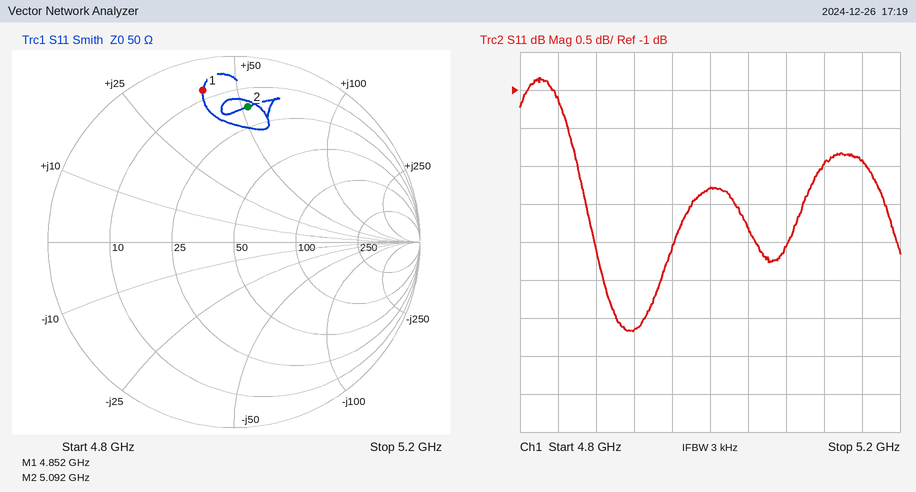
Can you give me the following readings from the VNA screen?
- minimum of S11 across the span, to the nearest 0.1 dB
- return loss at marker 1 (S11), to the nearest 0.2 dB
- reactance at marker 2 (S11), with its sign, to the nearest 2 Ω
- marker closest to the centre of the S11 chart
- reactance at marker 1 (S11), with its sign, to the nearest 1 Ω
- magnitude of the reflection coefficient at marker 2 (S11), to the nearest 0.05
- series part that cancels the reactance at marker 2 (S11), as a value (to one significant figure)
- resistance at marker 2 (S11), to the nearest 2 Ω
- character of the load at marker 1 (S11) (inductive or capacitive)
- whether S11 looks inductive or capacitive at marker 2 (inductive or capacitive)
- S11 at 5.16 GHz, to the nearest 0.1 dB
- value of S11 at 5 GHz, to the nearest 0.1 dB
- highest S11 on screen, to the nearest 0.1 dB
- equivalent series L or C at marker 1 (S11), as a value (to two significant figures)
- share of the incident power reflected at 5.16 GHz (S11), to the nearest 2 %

-4.2 dB
1.6 dB
+52 Ω
marker 2
+40 Ω
0.75
600 fF
16 Ω
inductive
inductive
-1.9 dB
-2.3 dB
-0.8 dB
1.3 nH
64 %
